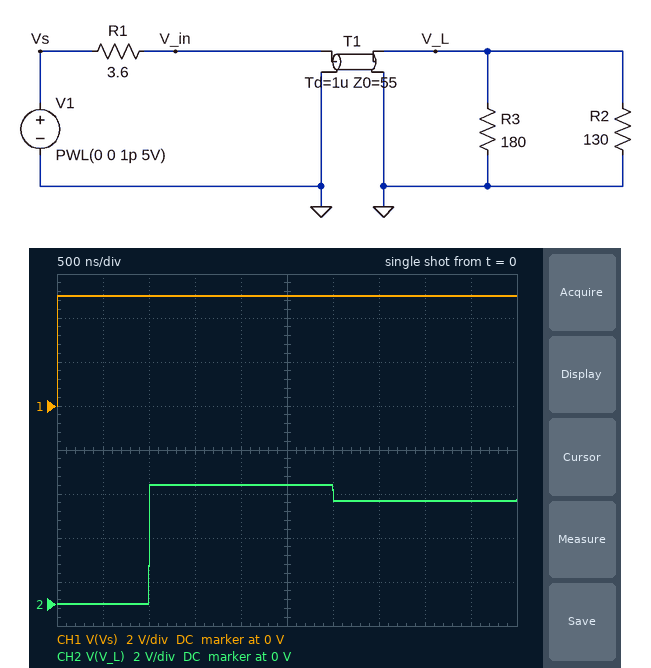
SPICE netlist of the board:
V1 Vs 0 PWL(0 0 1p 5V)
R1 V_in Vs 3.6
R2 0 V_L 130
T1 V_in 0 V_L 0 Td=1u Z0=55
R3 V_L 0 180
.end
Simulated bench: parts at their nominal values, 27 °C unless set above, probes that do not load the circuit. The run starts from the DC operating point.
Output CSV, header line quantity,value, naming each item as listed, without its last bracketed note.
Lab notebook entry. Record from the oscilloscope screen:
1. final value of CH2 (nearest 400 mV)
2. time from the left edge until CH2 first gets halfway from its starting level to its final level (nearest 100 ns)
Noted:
quantity,value
final value of CH2,4.8 V
time from the left edge until CH2 first gets halfway from its starting level to its final level,1.0 µs
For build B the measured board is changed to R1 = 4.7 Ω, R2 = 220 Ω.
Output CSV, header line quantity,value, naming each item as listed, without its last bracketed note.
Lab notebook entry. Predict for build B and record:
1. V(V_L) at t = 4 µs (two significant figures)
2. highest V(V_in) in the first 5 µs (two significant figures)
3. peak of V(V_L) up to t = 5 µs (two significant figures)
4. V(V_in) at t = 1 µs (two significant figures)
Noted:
quantity,value
V(V_L) at t = 4 µs,4.5 V
highest V(V_in) in the first 5 µs,4.8 V
peak of V(V_L) up to t = 5 µs,5.9 V
V(V_in) at t = 1 µs,4.6 V
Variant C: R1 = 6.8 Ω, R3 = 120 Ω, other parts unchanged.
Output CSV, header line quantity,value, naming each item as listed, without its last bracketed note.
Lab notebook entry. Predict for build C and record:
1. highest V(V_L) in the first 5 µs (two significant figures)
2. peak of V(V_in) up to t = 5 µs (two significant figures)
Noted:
quantity,value
highest V(V_L) in the first 5 µs,4.7 V
peak of V(V_in) up to t = 5 µs,4.5 V
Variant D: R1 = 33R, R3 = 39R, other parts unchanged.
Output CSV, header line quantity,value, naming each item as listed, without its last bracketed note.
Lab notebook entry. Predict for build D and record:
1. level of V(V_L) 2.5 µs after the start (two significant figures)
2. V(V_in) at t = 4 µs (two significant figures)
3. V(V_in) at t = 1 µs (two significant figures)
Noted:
quantity,value
level of V(V_L) 2.5 µs after the start,2.2 V
V(V_in) at t = 4 µs,2.4 V
V(V_in) at t = 1 µs,3.1 V
